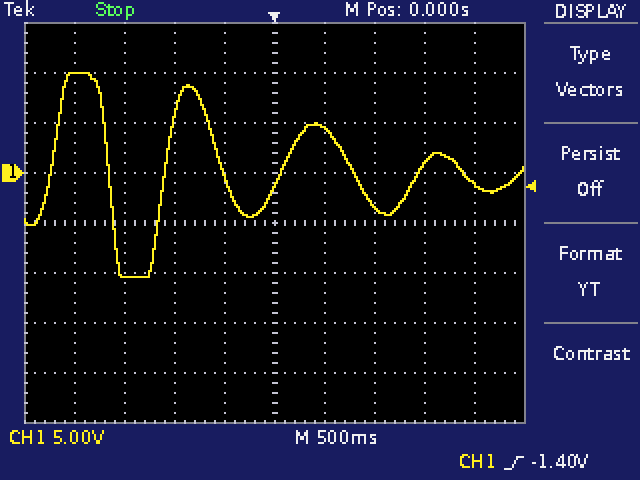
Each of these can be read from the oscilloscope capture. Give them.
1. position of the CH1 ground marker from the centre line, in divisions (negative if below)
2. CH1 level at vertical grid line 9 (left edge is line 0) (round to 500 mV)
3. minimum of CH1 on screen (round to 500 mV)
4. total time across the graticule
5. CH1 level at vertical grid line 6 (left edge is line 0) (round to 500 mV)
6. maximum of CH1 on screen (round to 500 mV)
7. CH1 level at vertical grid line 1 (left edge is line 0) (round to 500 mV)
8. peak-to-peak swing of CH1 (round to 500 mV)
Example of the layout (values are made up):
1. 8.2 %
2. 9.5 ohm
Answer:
1. +1.0 div
2. -1.0 V
3. -10.5 V
4. 5 s
5. 4.5 V
6. 10.0 V
7. 10.0 V
8. 20.5 V
